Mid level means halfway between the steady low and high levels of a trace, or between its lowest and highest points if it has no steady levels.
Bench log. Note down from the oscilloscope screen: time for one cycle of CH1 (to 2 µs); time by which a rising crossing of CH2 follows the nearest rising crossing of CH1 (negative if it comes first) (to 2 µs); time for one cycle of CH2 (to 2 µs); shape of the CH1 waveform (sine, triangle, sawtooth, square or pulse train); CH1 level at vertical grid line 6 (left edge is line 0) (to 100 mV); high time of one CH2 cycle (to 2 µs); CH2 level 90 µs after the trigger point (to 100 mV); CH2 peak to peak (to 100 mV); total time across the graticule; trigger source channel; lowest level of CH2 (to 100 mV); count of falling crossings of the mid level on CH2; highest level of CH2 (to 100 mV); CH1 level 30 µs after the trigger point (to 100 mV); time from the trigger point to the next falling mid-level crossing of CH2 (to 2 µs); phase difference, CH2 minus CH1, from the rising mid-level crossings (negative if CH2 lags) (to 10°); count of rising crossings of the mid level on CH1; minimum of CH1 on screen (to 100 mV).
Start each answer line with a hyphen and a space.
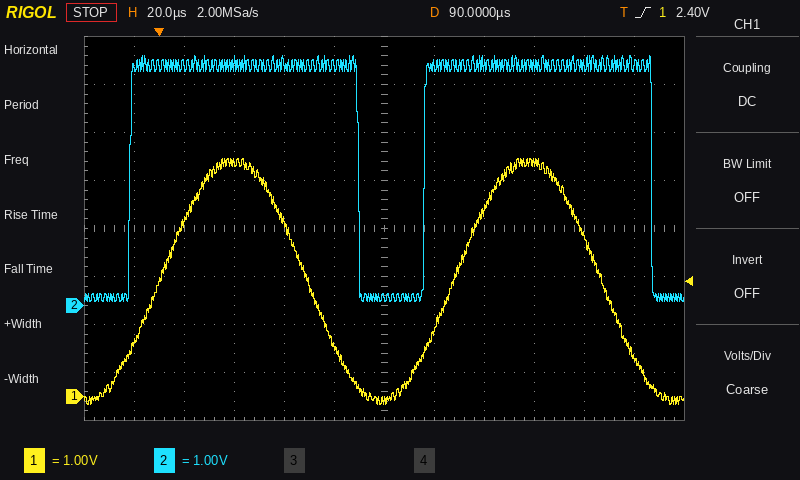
- 118 µs
- -12 µs
- 118 µs
- sine
- -100 mV
- 92 µs
- 200 mV
- 5.1 V
- 240 µs
- CH1
- 100 mV
- 2
- 5.2 V
- 4.9 V
- 80 µs
- +40°
- 2
- -200 mV
